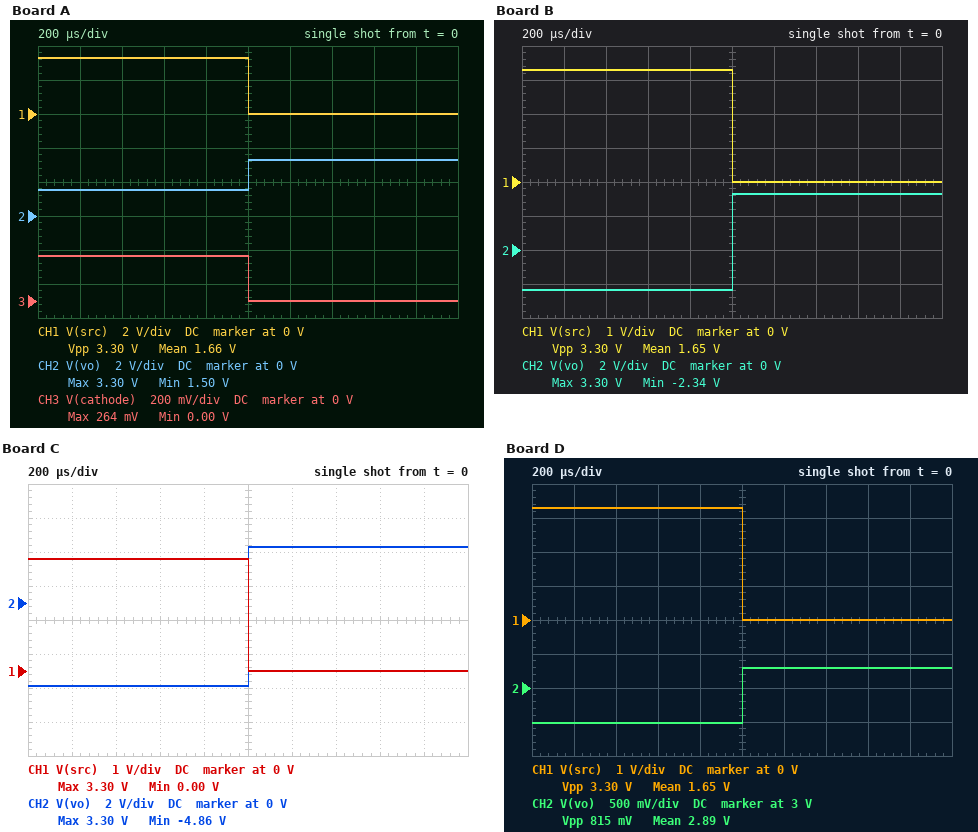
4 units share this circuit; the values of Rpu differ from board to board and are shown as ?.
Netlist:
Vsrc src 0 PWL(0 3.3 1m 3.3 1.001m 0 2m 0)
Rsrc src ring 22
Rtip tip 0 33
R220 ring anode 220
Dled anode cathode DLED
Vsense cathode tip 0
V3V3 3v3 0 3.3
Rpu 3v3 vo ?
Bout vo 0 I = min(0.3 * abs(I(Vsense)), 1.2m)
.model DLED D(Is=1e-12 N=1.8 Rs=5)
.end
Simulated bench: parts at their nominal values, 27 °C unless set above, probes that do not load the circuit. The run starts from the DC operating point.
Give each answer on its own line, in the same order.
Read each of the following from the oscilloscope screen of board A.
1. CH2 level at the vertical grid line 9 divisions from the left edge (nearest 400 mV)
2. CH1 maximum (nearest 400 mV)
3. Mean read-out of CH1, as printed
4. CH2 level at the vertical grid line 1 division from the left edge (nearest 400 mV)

3.2 V
3.2 V
1.66 V
1.6 V
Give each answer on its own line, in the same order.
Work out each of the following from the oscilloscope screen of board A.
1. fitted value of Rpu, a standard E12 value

1.5 kΩ
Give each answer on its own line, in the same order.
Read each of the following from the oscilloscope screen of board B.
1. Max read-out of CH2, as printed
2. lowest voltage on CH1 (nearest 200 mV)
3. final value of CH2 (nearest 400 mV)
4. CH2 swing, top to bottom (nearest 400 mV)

3.30 V
0 V
3.2 V
5.6 V
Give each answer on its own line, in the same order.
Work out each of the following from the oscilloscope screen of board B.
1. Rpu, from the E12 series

4.7 kΩ
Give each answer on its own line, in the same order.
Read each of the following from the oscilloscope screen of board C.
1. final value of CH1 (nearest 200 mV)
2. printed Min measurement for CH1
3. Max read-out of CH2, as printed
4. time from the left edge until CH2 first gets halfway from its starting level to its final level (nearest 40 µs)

0 V
0.00 V
3.30 V
1.00 ms
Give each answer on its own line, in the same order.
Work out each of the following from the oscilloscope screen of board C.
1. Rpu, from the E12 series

6.8 kΩ
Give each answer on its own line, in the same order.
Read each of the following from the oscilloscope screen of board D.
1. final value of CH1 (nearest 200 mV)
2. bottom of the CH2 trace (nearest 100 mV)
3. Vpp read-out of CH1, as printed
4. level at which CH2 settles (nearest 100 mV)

0 V
2.5 V
3.30 V
3.3 V
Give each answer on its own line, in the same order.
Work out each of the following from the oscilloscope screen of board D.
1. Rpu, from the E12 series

680 Ω
